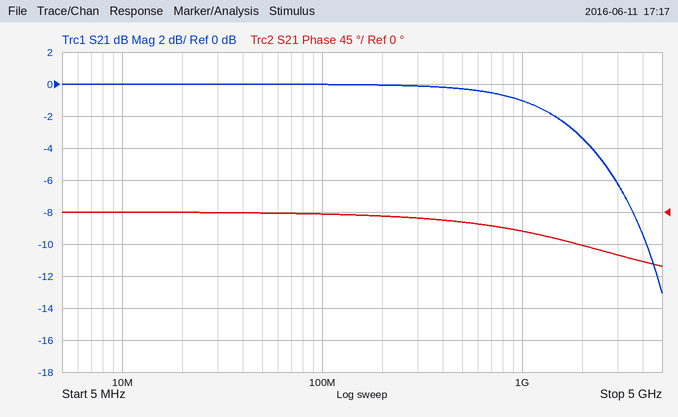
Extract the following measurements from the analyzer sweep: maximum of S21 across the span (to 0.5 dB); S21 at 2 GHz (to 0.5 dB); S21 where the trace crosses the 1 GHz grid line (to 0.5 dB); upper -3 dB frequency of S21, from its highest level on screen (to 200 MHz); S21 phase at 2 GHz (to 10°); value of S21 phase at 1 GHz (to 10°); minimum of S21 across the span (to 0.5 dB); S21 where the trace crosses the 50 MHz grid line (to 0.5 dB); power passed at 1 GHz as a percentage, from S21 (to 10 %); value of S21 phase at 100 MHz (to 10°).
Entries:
0.0 dB
-3.5 dB
-1.0 dB
1.8 GHz
-50°
-30°
-13.0 dB
0.0 dB
80 %
0°
